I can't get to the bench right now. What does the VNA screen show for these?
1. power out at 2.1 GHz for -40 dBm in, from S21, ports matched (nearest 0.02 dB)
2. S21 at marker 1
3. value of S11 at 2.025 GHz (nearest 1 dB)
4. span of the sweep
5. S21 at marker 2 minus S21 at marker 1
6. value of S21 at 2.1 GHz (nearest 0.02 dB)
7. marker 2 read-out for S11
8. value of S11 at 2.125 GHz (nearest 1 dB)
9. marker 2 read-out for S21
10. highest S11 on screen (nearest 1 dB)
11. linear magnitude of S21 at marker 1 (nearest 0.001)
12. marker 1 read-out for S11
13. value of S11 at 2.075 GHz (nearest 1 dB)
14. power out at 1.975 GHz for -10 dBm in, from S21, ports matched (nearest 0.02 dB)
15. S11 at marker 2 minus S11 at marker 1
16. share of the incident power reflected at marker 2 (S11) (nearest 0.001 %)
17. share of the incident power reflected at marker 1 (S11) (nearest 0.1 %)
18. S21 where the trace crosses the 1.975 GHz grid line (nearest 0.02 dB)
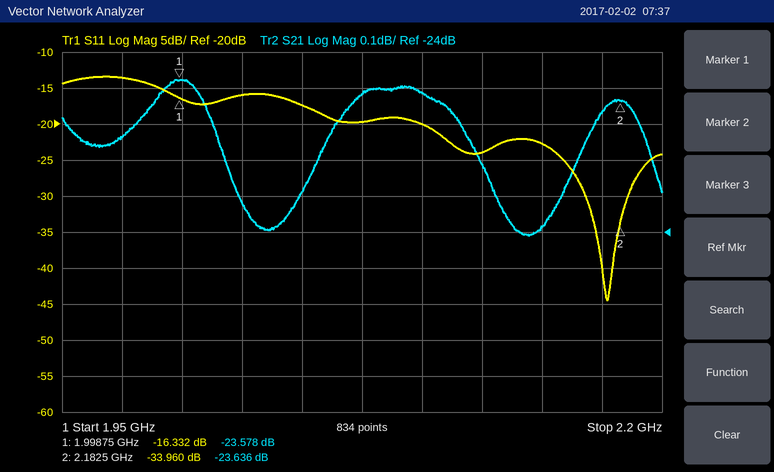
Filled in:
-63.62 dBm
-23.578 dB
-16 dB
250 MHz
-0.058 dB
-23.62 dB
-33.960 dB
-24 dB
-23.636 dB
-13 dB
0.066
-16.332 dB
-20 dB
-33.74 dBm
-17.628 dB
0.040 %
2.3 %
-23.74 dB
